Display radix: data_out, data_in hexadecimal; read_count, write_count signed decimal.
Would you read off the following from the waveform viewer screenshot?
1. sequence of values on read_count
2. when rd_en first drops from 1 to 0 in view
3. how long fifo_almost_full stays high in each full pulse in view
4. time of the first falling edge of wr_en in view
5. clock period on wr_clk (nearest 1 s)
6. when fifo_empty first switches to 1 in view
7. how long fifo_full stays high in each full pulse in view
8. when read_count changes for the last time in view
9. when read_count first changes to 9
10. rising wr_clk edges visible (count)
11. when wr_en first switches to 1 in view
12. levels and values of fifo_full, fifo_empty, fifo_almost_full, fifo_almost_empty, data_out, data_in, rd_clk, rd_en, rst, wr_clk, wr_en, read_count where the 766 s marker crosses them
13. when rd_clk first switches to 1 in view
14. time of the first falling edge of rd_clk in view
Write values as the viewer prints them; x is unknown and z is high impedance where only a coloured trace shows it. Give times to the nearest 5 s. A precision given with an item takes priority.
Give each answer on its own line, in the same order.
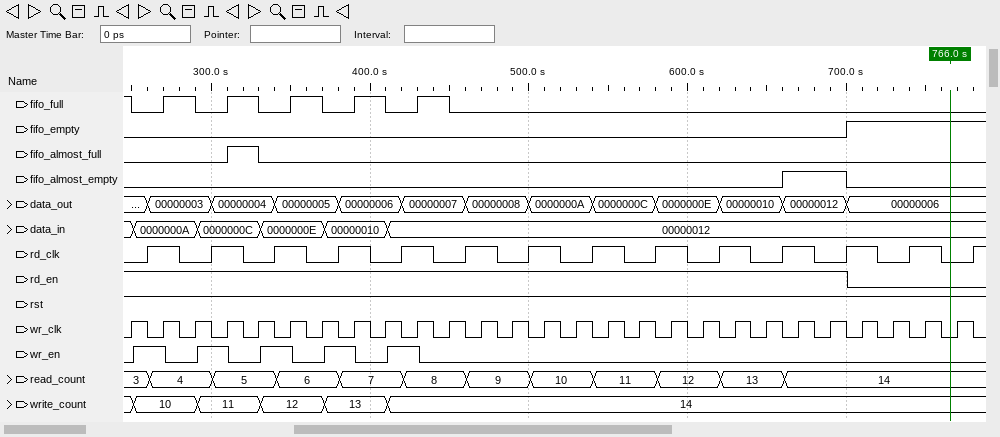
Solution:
3, 4, 5, 6, 7, 8, 9, 10, 11, 12, 13, 14
700 s
20 s
270 s
20 s
700 s
20 s, 20 s, 20 s, 20 s, 20 s
660 s
460 s
27
250 s
fifo_full=0, fifo_empty=1, fifo_almost_full=0, fifo_almost_empty=0, data_out=00000006, data_in=00000012, rd_clk=0, rd_en=0, rst=1, wr_clk=0, wr_en=0, read_count=14
260 s
280 s
